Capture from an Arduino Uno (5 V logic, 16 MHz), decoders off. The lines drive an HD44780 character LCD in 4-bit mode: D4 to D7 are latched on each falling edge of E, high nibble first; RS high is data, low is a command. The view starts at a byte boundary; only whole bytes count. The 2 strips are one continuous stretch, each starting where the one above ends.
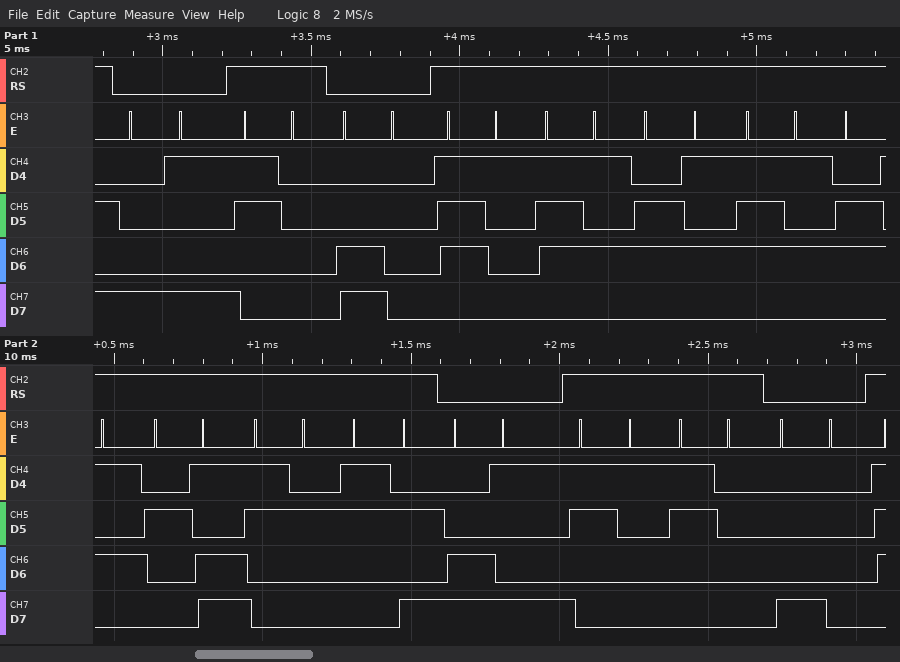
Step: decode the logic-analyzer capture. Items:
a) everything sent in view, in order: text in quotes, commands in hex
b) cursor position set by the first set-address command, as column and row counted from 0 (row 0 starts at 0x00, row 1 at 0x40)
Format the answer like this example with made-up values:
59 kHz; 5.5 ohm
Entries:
0x89 "0" 0xC0 "queue-2:" 0xC9 "10" 0x80; column 9, row 0
